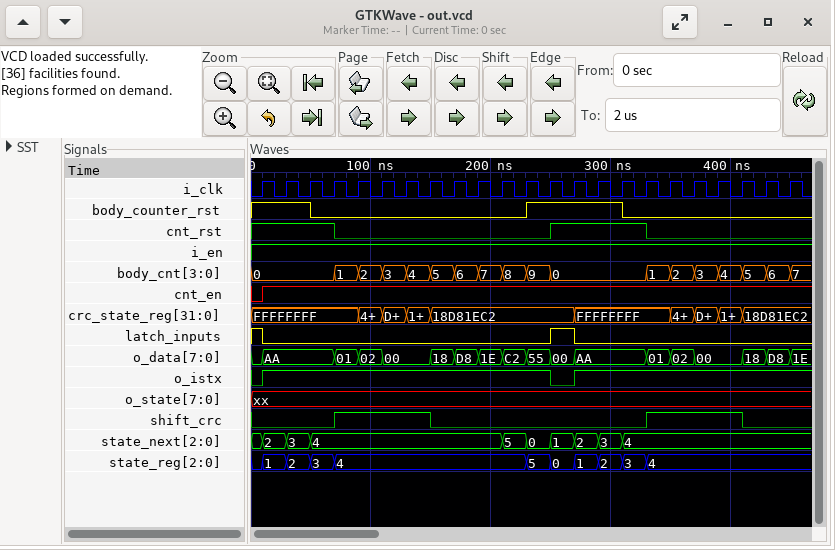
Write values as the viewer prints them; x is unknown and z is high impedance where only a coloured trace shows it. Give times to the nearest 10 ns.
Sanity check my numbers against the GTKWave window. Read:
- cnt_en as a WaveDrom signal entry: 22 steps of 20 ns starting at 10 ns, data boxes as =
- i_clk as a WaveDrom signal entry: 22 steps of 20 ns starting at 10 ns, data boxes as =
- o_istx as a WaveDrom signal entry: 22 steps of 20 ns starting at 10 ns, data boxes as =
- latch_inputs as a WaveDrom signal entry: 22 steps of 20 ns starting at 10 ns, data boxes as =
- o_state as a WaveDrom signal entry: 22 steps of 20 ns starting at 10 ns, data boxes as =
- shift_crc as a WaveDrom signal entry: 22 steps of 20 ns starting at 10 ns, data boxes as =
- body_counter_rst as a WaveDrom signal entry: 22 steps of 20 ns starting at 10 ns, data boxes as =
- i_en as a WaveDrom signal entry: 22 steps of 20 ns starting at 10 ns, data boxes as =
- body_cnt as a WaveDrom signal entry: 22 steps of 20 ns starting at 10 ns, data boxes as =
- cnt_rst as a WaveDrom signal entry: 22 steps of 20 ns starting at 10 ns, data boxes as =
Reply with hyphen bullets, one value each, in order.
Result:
- {name: 'cnt_en', wave: '1.....................'}
- {name: 'i_clk', wave: 'p.....................'}
- {name: 'o_istx', wave: '1...........01........'}
- {name: 'latch_inputs', wave: '0...........10........'}
- {name: 'o_state', wave: 'x.....................'}
- {name: 'shift_crc', wave: '0..1...0........1...0.'}
- {name: 'body_counter_rst', wave: '1.0........1...0......'}
- {name: 'i_en', wave: '1.....................'}
- {name: 'body_cnt', wave: '=..==========...======', data: '0 1 2 3 4 5 6 7 8 9 0 1 2 3 4 5 6'}
- {name: 'cnt_rst', wave: '1..0........1...0.....'}
